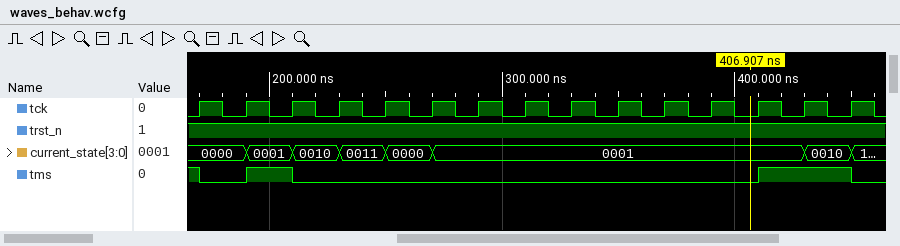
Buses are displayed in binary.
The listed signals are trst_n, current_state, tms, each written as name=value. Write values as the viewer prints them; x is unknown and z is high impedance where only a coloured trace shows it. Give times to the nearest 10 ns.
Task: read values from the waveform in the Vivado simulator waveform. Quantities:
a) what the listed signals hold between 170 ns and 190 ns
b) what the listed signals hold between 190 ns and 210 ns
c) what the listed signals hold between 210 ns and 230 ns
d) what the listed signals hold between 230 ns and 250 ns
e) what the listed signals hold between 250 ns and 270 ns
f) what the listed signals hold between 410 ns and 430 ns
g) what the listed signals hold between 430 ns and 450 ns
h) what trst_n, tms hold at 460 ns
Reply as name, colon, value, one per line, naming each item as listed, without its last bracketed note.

what the listed signals hold between 170 ns and 190 ns: trst_n=1, current_state=0000, tms=0
what the listed signals hold between 190 ns and 210 ns: trst_n=1, current_state=0001, tms=1
what the listed signals hold between 210 ns and 230 ns: trst_n=1, current_state=0010, tms=0
what the listed signals hold between 230 ns and 250 ns: trst_n=1, current_state=0011, tms=0
what the listed signals hold between 250 ns and 270 ns: trst_n=1, current_state=0000, tms=0
what the listed signals hold between 410 ns and 430 ns: trst_n=1, current_state=0001, tms=1
what the listed signals hold between 430 ns and 450 ns: trst_n=1, current_state=0010, tms=1
what trst_n, tms hold at 460 ns: trst_n=1, tms=0
